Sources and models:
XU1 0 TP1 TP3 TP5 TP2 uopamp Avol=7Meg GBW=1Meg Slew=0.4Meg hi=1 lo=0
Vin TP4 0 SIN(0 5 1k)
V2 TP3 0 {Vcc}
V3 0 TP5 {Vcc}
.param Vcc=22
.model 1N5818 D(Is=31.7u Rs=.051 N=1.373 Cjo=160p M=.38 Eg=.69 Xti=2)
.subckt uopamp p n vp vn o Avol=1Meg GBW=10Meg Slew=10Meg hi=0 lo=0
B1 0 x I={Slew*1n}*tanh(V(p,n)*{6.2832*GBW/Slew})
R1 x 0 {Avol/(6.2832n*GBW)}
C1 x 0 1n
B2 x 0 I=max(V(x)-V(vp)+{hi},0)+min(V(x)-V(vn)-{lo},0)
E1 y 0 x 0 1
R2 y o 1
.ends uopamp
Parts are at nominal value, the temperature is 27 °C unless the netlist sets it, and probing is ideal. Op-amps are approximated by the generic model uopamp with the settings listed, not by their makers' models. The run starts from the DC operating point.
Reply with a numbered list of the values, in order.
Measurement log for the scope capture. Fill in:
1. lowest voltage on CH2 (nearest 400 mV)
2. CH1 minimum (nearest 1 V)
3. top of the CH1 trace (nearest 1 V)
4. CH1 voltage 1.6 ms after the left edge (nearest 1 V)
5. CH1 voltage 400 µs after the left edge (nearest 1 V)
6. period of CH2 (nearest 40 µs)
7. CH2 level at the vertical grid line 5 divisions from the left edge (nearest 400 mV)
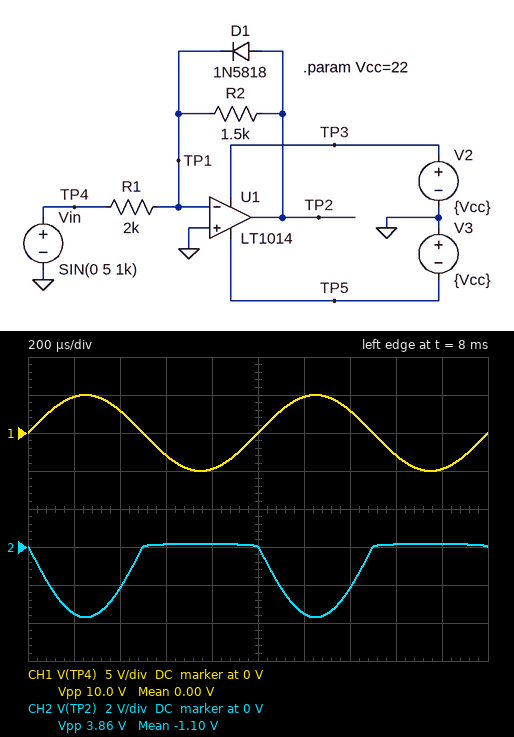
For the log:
1. -3.6 V
2. -5 V
3. 5 V
4. -3 V
5. 3 V
6. 1.00 ms
7. 0 V
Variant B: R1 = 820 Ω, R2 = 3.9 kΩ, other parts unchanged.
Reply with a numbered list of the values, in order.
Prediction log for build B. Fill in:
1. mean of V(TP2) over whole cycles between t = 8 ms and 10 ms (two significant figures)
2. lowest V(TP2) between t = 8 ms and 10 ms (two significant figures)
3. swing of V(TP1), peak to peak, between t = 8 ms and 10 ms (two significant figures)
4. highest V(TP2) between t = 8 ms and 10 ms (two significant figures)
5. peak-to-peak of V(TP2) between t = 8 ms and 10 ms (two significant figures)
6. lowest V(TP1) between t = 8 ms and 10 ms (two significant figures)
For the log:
1. -7.3 V
2. -22 V
3. 310 mV
4. 190 mV
5. 22 V
6. -25 mV
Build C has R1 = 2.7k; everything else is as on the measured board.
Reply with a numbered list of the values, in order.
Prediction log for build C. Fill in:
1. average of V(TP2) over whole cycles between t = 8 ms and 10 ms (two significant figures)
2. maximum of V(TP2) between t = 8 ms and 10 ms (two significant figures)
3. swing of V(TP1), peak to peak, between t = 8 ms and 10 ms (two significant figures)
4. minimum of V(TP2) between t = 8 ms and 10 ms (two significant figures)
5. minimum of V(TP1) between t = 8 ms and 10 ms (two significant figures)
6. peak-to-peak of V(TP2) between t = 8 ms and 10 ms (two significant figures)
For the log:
1. -800 mV
2. 140 mV
3. 5.5 mV
4. -2.7 V
5. -2.8 mV
6. 2.9 V
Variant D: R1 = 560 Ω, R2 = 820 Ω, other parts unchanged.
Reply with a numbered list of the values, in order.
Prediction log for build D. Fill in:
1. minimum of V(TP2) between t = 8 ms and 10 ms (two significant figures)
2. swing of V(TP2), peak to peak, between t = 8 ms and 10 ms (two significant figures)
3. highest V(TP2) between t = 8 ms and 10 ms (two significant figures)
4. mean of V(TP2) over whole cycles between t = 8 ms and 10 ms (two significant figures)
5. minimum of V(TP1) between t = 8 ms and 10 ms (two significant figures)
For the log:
1. -7.3 V
2. 7.5 V
3. 200 mV
4. -2.2 V
5. -7.3 mV
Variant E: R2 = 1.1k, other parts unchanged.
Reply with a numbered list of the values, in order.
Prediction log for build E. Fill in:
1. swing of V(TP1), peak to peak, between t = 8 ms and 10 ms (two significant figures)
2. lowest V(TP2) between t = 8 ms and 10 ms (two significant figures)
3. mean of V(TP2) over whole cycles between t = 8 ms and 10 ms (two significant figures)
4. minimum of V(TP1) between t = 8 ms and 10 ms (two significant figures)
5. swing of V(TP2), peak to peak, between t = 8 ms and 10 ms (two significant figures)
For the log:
1. 5.5 mV
2. -2.7 V
3. -790 mV
4. -2.7 mV
5. 2.9 V
